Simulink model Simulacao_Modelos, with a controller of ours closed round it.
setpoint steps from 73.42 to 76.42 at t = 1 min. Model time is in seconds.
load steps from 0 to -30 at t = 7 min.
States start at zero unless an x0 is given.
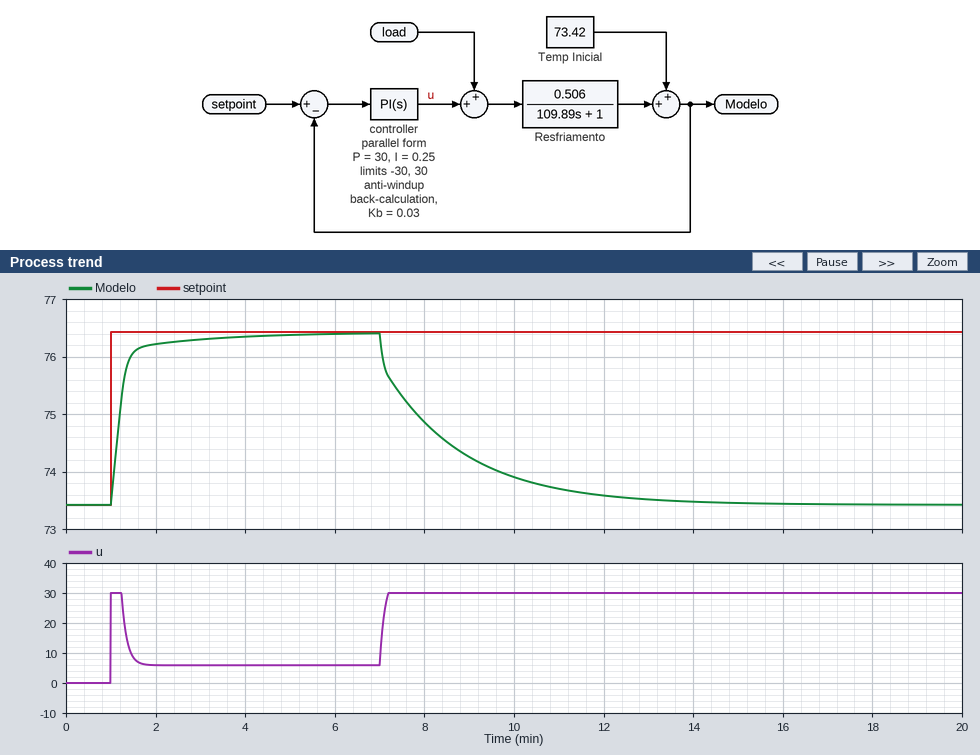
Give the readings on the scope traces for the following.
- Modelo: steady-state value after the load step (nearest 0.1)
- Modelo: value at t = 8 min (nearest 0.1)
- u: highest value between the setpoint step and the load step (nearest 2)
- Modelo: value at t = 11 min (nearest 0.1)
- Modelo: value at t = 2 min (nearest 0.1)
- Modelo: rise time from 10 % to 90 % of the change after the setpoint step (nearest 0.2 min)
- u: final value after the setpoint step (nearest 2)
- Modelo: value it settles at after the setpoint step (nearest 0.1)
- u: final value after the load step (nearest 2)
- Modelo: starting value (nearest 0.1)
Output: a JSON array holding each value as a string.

["73.4", "74.9", "30", "73.7", "76.2", "0.6 min", "6", "76.4", "30", "73.4"]
